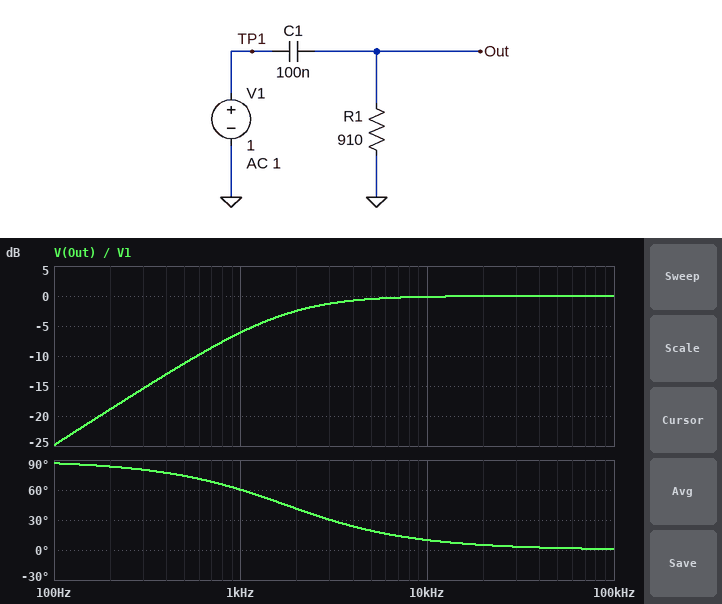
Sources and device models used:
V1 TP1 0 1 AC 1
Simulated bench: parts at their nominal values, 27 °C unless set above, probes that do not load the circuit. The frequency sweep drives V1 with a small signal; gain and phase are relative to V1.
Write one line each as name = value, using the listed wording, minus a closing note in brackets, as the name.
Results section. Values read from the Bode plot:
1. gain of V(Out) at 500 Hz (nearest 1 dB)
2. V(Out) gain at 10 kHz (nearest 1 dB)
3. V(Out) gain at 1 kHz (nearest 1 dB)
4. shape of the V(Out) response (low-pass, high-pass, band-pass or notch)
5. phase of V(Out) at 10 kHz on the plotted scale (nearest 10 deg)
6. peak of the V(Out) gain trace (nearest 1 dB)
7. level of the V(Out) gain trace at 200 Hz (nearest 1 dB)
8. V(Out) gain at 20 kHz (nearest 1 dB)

gain of V(Out) at 500 Hz = -11 dB
V(Out) gain at 10 kHz = 0 dB
V(Out) gain at 1 kHz = -6 dB
shape of the V(Out) response = high-pass
phase of V(Out) at 10 kHz on the plotted scale = 10 deg
peak of the V(Out) gain trace = 0 dB
level of the V(Out) gain trace at 200 Hz = -19 dB
V(Out) gain at 20 kHz = 0 dB
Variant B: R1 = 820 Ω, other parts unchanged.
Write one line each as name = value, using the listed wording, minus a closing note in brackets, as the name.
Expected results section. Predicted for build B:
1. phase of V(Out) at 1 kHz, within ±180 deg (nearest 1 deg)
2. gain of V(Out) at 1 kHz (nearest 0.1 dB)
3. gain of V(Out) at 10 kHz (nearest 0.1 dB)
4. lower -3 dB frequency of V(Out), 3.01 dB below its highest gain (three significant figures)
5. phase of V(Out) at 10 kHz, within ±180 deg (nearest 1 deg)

phase of V(Out) at 1 kHz, within ±180 deg = 63 deg
gain of V(Out) at 1 kHz = -6.8 dB
gain of V(Out) at 10 kHz = -0.2 dB
lower -3 dB frequency of V(Out), 3.01 dB below its highest gain = 1.94 kHz
phase of V(Out) at 10 kHz, within ±180 deg = 11 deg
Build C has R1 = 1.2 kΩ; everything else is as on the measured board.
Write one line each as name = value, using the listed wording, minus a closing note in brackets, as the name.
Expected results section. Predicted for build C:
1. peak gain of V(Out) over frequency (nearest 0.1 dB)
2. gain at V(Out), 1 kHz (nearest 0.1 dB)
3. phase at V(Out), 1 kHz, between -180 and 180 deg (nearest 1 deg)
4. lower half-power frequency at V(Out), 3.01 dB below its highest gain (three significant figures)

peak gain of V(Out) over frequency = 0 dB
gain at V(Out), 1 kHz = -4.4 dB
phase at V(Out), 1 kHz, between -180 and 180 deg = 53 deg
lower half-power frequency at V(Out), 3.01 dB below its highest gain = 1.33 kHz
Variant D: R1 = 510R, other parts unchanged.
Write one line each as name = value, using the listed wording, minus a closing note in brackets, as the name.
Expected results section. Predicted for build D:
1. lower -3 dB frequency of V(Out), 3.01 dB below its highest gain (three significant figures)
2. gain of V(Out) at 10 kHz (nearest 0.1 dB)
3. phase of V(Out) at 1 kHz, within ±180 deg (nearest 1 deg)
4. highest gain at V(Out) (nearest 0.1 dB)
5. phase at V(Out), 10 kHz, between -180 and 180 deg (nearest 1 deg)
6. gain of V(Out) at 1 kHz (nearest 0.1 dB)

lower -3 dB frequency of V(Out), 3.01 dB below its highest gain = 3.12 kHz
gain of V(Out) at 10 kHz = -0.4 dB
phase of V(Out) at 1 kHz, within ±180 deg = 72 deg
highest gain at V(Out) = 0 dB
phase at V(Out), 10 kHz, between -180 and 180 deg = 17 deg
gain of V(Out) at 1 kHz = -10.3 dB
